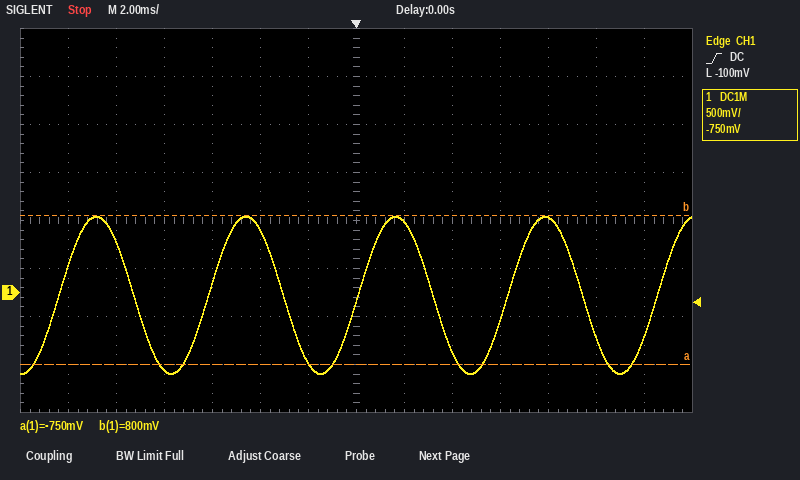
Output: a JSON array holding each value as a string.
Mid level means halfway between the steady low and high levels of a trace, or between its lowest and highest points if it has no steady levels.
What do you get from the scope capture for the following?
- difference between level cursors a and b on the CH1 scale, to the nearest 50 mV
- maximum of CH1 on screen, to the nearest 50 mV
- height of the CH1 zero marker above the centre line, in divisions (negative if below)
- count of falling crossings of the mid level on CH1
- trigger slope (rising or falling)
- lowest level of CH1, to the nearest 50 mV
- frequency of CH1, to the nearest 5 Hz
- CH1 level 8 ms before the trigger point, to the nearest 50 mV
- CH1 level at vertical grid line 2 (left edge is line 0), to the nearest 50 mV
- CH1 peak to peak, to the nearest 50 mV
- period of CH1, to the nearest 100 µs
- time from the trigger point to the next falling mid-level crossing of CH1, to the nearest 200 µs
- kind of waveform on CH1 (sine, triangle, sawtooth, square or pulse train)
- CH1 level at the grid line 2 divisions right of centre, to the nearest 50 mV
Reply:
["1.55 V", "800 mV", "-1.5 div", "4", "rising", "-850 mV", "160 Hz", "-800 mV", "550 mV", "1.65 V", "6.2 ms", "3.2 ms", "sine", "-600 mV"]
